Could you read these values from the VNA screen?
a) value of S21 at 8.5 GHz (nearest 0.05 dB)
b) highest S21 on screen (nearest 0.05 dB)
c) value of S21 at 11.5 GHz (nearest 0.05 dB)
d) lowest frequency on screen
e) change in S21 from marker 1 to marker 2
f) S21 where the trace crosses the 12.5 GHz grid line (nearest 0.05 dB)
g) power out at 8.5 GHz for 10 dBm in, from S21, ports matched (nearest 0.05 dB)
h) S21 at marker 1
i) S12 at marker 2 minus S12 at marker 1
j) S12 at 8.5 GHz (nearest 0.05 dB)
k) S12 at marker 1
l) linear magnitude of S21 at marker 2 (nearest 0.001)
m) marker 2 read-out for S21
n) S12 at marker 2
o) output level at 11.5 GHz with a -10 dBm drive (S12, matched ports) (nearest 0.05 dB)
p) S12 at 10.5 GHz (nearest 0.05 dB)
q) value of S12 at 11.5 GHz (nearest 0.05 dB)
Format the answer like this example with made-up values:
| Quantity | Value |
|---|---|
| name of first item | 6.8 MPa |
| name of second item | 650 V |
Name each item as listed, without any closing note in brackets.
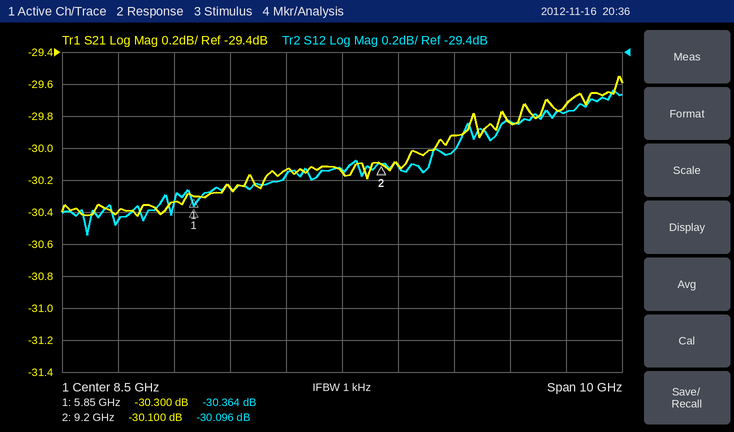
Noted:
| Quantity | Value |
|---|---|
| value of S21 at 8.5 GHz | -30.15 dB |
| highest S21 on screen | -29.55 dB |
| value of S21 at 11.5 GHz | -29.85 dB |
| lowest frequency on screen | 3.5 GHz |
| change in S21 from marker 1 to marker 2 | 0.200 dB |
| S21 where the trace crosses the 12.5 GHz grid line | -29.75 dB |
| power out at 8.5 GHz for 10 dBm in, from S21, ports matched | -20.15 dBm |
| S21 at marker 1 | -30.300 dB |
| S12 at marker 2 minus S12 at marker 1 | 0.268 dB |
| S12 at 8.5 GHz | -30.15 dB |
| S12 at marker 1 | -30.364 dB |
| linear magnitude of S21 at marker 2 | 0.031 |
| marker 2 read-out for S21 | -30.100 dB |
| S12 at marker 2 | -30.096 dB |
| output level at 11.5 GHz with a -10 dBm drive (S12, matched ports) | -39.85 dBm |
| S12 at 10.5 GHz | -30.00 dB |
| value of S12 at 11.5 GHz | -29.85 dB |
